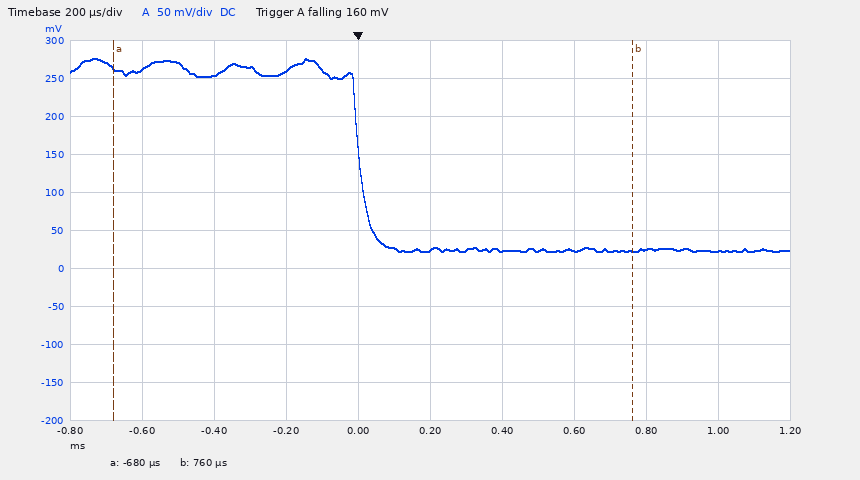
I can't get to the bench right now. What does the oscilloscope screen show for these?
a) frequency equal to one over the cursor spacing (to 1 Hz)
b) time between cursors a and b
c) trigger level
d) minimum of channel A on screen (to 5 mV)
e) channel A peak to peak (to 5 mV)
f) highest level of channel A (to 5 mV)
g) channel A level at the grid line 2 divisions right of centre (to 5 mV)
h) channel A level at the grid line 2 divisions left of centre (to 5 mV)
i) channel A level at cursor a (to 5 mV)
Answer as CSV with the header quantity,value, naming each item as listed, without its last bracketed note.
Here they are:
quantity,value
frequency equal to one over the cursor spacing,694 Hz
time between cursors a and b,1.44 ms
trigger level,160 mV
minimum of channel A on screen,20 mV
channel A peak to peak,255 mV
highest level of channel A,275 mV
channel A level at the grid line 2 divisions right of centre,25 mV
channel A level at the grid line 2 divisions left of centre,260 mV
channel A level at cursor a,265 mV
